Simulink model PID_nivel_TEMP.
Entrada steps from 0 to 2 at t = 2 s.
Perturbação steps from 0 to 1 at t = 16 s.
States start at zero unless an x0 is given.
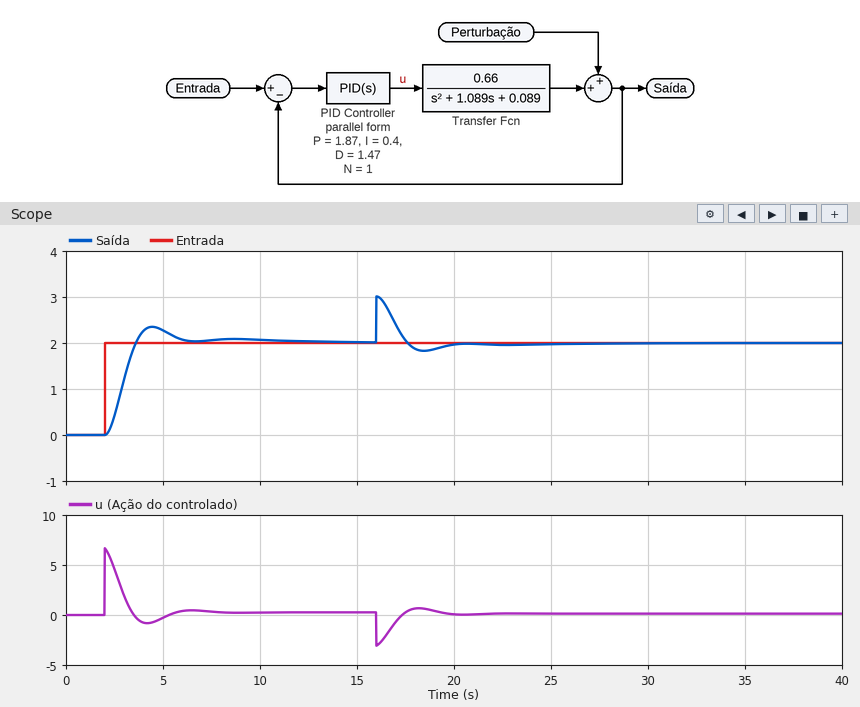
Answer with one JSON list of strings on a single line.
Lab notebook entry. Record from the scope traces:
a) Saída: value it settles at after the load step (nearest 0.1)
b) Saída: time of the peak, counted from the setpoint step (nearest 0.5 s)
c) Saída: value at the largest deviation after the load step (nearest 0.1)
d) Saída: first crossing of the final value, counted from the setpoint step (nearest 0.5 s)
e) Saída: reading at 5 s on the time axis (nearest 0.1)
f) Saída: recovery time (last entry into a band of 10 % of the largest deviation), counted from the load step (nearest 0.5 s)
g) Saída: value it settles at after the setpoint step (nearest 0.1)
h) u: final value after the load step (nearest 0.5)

["2.0", "2.5 s", "3.0", "1.5 s", "2.3", "3.5 s", "2.0", "0.0"]
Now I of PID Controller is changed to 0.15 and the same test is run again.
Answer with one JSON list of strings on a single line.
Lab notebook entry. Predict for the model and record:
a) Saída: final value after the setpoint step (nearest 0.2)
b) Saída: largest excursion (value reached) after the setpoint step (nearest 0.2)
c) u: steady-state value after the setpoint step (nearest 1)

["2.0", "2.2", "0"]
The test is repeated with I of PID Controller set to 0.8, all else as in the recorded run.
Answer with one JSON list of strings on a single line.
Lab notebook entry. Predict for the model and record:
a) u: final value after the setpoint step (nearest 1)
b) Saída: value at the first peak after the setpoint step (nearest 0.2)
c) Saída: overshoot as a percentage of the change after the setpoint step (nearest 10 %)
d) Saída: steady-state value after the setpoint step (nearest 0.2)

["0", "2.6", "30 %", "2.0"]
